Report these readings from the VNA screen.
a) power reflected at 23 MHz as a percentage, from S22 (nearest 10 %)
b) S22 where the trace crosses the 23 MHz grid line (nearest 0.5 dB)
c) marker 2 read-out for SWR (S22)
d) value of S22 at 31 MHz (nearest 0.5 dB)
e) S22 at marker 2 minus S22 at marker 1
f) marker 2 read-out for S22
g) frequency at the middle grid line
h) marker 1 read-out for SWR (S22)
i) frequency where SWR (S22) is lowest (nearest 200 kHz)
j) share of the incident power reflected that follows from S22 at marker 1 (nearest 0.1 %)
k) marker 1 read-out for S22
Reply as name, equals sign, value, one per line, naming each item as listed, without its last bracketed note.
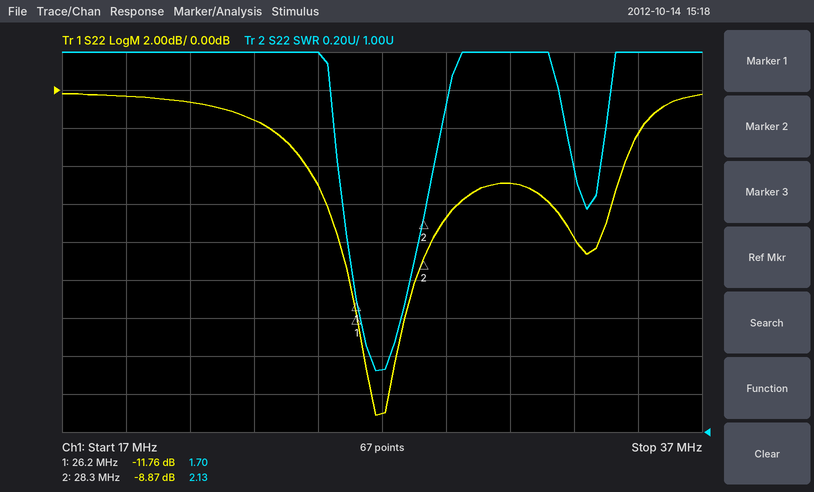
power reflected at 23 MHz as a percentage, from S22 = 70 %
S22 where the trace crosses the 23 MHz grid line = -1.5 dB
marker 2 read-out for SWR = 2.13
value of S22 at 31 MHz = -5.0 dB
S22 at marker 2 minus S22 at marker 1 = 2.89 dB
marker 2 read-out for S22 = -8.87 dB
frequency at the middle grid line = 27 MHz
marker 1 read-out for SWR = 1.70
frequency where SWR (S22) is lowest = 26.8 MHz
share of the incident power reflected that follows from S22 at marker 1 = 6.7 %
marker 1 read-out for S22 = -11.76 dB
